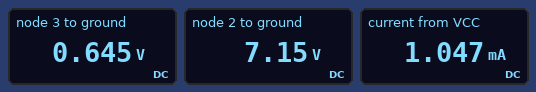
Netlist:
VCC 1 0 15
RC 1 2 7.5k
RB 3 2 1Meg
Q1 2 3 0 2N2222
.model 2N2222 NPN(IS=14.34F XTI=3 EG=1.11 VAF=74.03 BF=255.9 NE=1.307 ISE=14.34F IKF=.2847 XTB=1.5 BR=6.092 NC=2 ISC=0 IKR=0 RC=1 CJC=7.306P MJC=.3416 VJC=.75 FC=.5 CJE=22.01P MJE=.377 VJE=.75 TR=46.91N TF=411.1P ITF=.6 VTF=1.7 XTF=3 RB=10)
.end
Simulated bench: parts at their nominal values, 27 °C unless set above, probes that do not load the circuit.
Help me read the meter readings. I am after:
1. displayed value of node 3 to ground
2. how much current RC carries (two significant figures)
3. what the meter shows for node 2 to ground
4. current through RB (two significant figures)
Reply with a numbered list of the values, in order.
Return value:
1. 0.645 V
2. 1.0 mA
3. 7.15 V
4. 6.5 µA
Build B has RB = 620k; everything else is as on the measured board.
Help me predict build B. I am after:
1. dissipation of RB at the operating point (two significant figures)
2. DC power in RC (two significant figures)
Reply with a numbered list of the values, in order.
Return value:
1. 38 µW
2. 12 mW
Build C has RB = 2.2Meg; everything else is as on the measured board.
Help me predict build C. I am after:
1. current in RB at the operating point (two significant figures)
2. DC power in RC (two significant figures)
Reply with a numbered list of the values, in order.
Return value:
1. 4.2 µA
2. 3.4 mW
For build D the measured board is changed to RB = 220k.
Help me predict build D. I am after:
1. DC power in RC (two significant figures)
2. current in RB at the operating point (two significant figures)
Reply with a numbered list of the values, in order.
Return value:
1. 20 mW
2. 10 µA
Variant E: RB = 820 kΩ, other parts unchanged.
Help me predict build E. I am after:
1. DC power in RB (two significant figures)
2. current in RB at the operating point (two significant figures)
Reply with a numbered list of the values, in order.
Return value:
1. 41 µW
2. 7.1 µA
